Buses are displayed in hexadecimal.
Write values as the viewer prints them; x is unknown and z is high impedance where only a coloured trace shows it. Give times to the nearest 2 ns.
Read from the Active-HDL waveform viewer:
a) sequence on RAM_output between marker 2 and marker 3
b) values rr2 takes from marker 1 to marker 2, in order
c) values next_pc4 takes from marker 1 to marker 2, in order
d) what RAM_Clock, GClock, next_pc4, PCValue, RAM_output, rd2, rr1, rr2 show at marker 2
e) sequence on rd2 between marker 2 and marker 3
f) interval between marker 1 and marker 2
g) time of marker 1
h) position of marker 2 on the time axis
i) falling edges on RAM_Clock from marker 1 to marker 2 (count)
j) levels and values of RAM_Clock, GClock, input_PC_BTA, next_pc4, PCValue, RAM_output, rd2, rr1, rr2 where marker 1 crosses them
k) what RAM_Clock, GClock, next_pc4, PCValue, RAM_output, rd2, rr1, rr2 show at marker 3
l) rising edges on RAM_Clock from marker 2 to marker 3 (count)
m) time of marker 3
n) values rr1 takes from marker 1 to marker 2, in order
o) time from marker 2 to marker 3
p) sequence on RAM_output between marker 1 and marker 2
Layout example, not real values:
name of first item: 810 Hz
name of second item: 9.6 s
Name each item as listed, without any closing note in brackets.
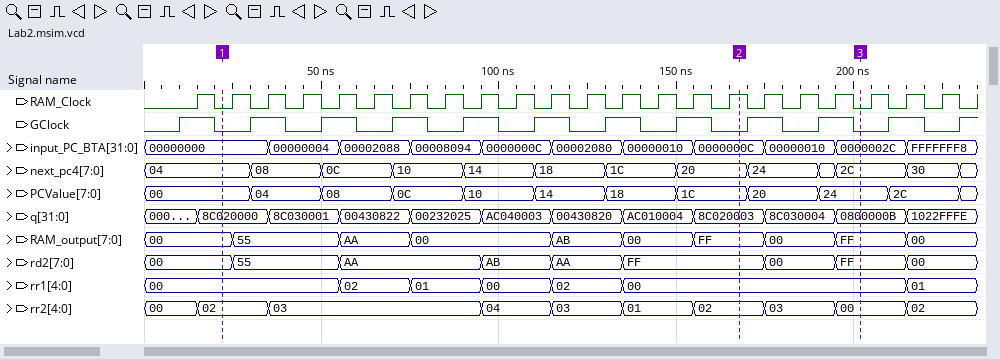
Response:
sequence on RAM_output between marker 2 and marker 3: FF, 00, FF
values rr2 takes from marker 1 to marker 2, in order: 02, 03, 04, 03, 01, 02
values next_pc4 takes from marker 1 to marker 2, in order: 04, 08, 0C, 10, 14, 18, 1C, 20
what RAM_Clock, GClock, next_pc4, PCValue, RAM_output, rd2, rr1, rr2 show at marker 2: RAM_Clock=1, GClock=0, next_pc4=20, PCValue=1C, RAM_output=FF, rd2=FF, rr1=00, rr2=02
sequence on rd2 between marker 2 and marker 3: FF, 00, FF
interval between marker 1 and marker 2: 146 ns
time of marker 1: 22 ns
position of marker 2 on the time axis: 168 ns
falling edges on RAM_Clock from marker 1 to marker 2: 14
levels and values of RAM_Clock, GClock, input_PC_BTA, next_pc4, PCValue, RAM_output, rd2, rr1, rr2 where marker 1 crosses them: RAM_Clock=0, GClock=0, input_PC_BTA=00000000, next_pc4=04, PCValue=00, RAM_output=00, rd2=00, rr1=00, rr2=02
what RAM_Clock, GClock, next_pc4, PCValue, RAM_output, rd2, rr1, rr2 show at marker 3: RAM_Clock=0, GClock=0, next_pc4=2C, PCValue=24, RAM_output=FF, rd2=FF, rr1=00, rr2=00
rising edges on RAM_Clock from marker 2 to marker 3: 3
time of marker 3: 202 ns
values rr1 takes from marker 1 to marker 2, in order: 00, 02, 01, 00, 02, 00
time from marker 2 to marker 3: 34 ns
sequence on RAM_output between marker 1 and marker 2: 00, 55, AA, 00, AB, 00, FF
